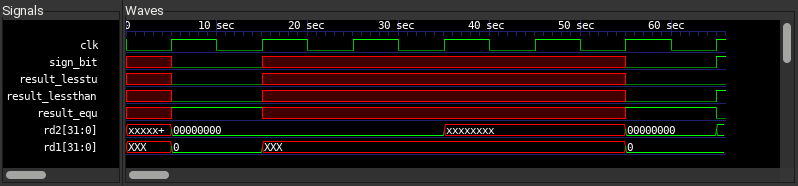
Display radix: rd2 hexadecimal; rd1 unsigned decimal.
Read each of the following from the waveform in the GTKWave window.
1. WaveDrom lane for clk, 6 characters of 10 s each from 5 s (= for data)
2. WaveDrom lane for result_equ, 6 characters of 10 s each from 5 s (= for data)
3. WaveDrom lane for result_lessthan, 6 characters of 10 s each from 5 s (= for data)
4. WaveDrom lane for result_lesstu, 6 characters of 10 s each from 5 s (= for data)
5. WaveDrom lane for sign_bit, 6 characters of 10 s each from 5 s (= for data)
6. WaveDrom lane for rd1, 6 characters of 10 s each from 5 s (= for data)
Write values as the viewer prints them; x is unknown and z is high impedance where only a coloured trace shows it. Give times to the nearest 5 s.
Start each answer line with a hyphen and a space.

- {name: 'clk', wave: 'p.....'}
- {name: 'result_equ', wave: '1x...1'}
- {name: 'result_lessthan', wave: '0x...0'}
- {name: 'result_lesstu', wave: '0x...0'}
- {name: 'sign_bit', wave: '0x...0'}
- {name: 'rd1', wave: '=x...=', data: '0 0'}
